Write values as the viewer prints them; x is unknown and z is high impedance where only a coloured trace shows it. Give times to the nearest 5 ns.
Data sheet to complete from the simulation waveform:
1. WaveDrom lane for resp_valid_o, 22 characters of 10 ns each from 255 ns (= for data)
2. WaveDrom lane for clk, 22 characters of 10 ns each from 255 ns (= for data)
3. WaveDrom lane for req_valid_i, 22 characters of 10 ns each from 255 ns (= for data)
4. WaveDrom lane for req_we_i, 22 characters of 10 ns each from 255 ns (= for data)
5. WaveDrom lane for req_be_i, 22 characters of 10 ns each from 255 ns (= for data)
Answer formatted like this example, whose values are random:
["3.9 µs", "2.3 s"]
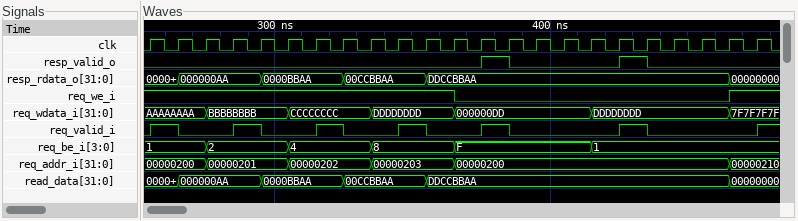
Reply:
["{name: 'resp_valid_o', wave: '0...........10...10...'}", "{name: 'clk', wave: 'p.....................'}", "{name: 'req_valid_i', wave: '10.10.10.10.10...10...'}", "{name: 'req_we_i', wave: '1..........0.........1'}", "{name: 'req_be_i', wave: '=.=..=..=..=....=.....', data: '1 2 4 8 F 1'}"]
